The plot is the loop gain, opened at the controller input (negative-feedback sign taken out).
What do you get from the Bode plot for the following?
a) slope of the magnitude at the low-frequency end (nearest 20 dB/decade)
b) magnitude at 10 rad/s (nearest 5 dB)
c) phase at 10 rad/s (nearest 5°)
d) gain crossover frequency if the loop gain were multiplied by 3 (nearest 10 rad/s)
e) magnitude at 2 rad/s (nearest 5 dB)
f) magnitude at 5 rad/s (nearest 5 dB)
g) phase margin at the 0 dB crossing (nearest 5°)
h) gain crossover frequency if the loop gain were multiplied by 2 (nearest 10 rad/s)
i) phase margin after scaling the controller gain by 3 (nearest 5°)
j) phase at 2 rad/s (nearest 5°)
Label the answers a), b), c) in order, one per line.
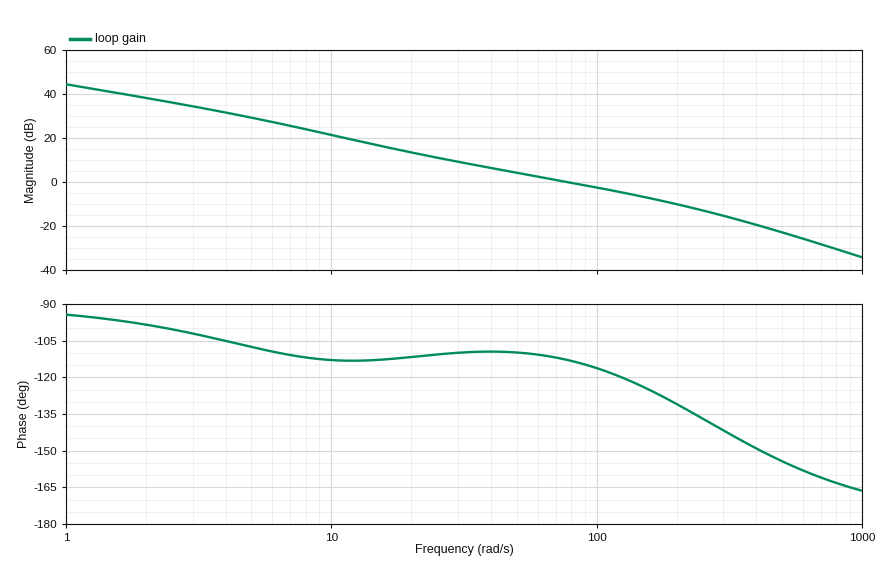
a) -20 dB/decade
b) 20 dB
c) -115°
d) 190 rad/s
e) 40 dB
f) 30 dB
g) 65°
h) 140 rad/s
i) 50°
j) -100°
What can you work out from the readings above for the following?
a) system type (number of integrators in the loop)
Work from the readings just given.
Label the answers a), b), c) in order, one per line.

a) 1
